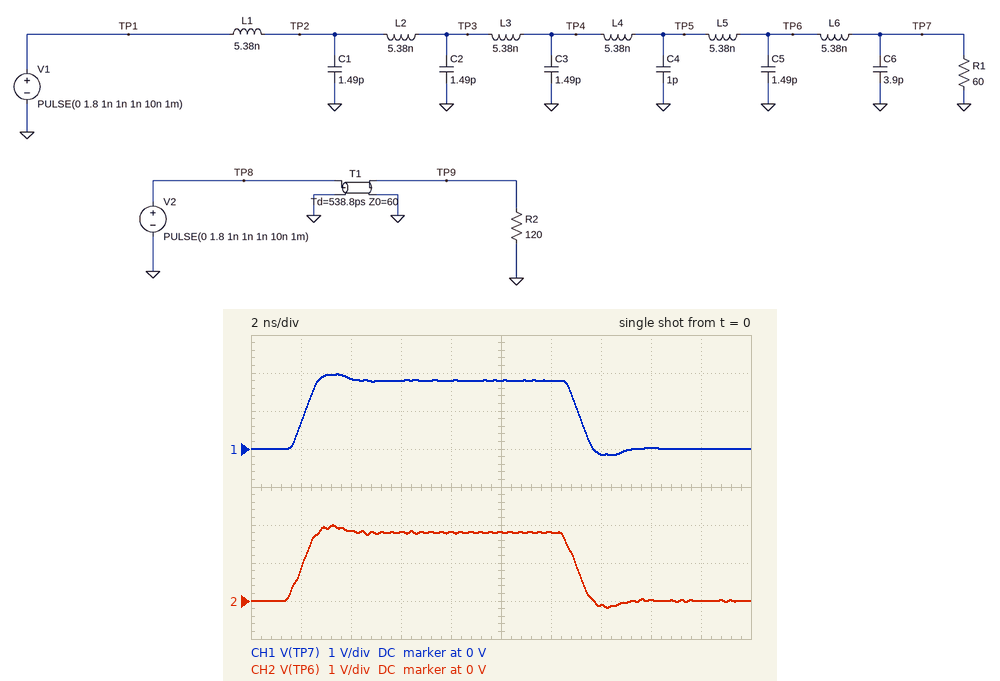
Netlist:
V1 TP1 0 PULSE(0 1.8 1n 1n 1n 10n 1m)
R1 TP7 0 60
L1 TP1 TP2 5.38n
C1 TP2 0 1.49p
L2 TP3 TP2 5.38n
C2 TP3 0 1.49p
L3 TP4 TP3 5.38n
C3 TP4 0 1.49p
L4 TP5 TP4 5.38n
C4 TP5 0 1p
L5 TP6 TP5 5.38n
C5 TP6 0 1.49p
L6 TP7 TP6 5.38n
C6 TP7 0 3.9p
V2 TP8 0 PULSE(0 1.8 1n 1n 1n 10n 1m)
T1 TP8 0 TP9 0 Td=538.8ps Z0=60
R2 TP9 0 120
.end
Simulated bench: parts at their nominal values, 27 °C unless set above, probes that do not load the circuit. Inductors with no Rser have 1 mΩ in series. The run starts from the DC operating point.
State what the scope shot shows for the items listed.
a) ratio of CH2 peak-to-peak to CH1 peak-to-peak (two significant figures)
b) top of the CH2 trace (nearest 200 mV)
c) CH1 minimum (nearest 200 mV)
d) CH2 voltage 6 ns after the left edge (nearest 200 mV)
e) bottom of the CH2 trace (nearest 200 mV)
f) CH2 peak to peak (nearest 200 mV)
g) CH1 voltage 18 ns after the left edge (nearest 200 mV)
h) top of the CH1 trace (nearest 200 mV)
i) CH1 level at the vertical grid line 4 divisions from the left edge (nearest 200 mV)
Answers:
1.0
2.0 V
-200 mV
1.8 V
-200 mV
2.2 V
0 V
2.0 V
1.8 V
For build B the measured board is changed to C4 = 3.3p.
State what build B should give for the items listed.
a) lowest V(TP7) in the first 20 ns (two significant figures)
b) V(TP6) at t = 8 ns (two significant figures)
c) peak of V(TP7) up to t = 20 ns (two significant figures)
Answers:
-260 mV
1.8 V
2.1 V
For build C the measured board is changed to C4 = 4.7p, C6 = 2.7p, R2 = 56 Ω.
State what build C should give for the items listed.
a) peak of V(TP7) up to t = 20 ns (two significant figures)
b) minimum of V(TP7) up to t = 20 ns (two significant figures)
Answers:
2.1 V
-270 mV
